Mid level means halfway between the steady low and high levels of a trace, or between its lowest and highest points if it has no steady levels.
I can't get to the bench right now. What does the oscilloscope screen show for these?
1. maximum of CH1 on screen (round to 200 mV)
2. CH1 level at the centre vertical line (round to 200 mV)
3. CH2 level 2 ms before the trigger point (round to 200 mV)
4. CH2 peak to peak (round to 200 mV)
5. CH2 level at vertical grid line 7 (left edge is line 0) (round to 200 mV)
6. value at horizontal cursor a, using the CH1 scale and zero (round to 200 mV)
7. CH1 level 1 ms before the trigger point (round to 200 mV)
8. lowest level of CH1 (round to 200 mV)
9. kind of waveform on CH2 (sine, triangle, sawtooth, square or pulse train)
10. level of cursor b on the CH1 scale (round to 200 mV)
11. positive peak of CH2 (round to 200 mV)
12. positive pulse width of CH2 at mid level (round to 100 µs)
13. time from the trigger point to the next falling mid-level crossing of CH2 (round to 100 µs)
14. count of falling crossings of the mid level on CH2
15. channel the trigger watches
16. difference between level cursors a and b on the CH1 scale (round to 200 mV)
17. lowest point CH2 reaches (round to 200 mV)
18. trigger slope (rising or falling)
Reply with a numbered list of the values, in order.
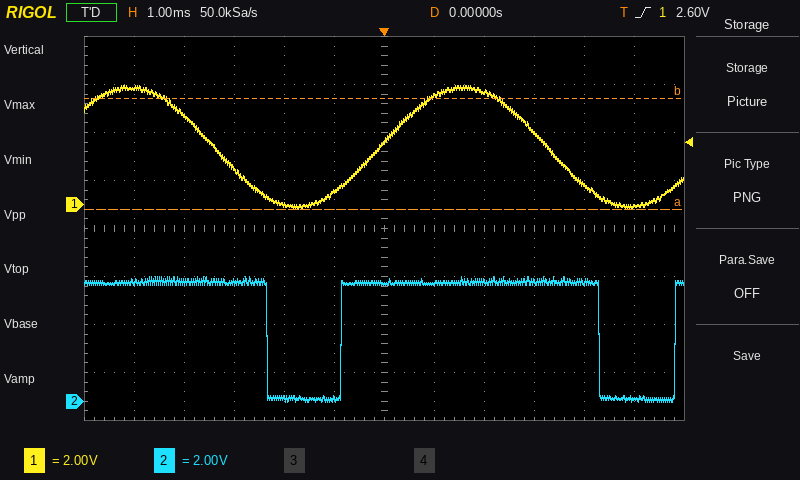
1. 5.0 V
2. 2.6 V
3. 200 mV
4. 5.2 V
5. 5.0 V
6. -200 mV
7. 600 mV
8. -200 mV
9. pulse train
10. 4.4 V
11. 5.2 V
12. 5.2 ms
13. 4.3 ms
14. 2
15. CH1
16. 4.6 V
17. 0.0 V
18. rising
